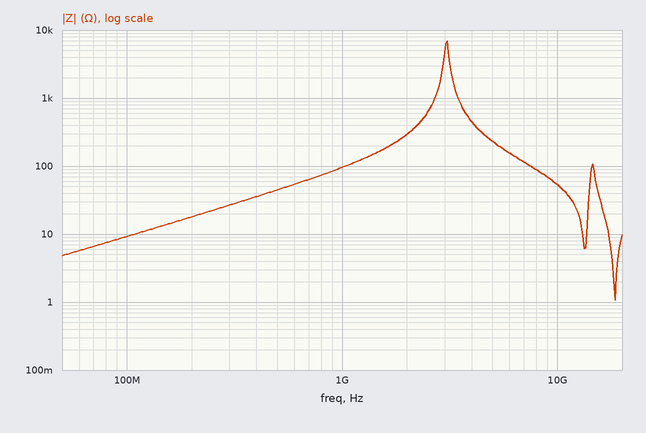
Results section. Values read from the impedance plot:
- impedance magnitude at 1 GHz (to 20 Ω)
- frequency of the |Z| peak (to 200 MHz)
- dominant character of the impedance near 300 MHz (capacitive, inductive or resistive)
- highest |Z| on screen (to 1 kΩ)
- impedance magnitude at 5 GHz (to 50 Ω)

100 Ω
3.0 GHz
inductive
7 kΩ
250 Ω
